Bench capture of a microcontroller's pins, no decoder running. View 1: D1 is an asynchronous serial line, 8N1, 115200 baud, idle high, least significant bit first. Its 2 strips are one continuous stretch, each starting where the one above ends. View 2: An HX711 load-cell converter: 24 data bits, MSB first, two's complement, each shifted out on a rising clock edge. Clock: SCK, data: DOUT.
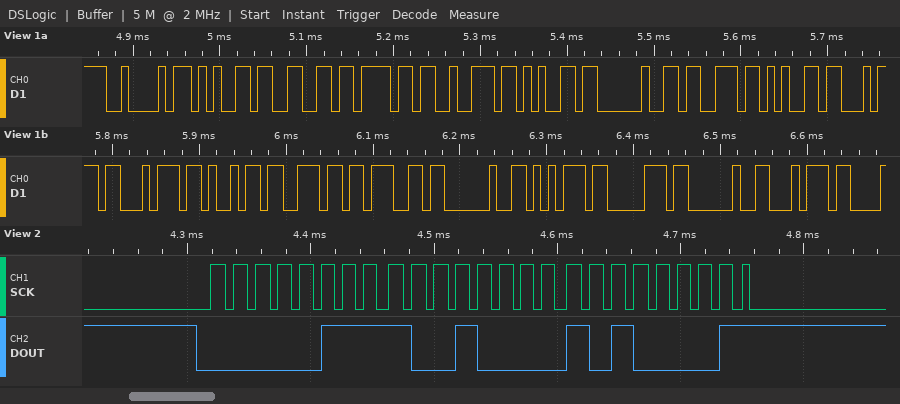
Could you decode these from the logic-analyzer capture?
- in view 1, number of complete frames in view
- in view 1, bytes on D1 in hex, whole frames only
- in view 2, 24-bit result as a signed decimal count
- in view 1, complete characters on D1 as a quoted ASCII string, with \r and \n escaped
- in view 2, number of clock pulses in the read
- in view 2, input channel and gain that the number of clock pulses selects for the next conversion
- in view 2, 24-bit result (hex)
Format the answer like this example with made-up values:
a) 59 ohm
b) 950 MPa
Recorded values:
a) 19
b) 42 65 66 6F 72 65 20 73 65 74 74 69 6E 67 20 75 70 20 74
c) 495777
d) "Before setting up t"
e) 25
f) channel A, gain 128
g) 0x0790A1
